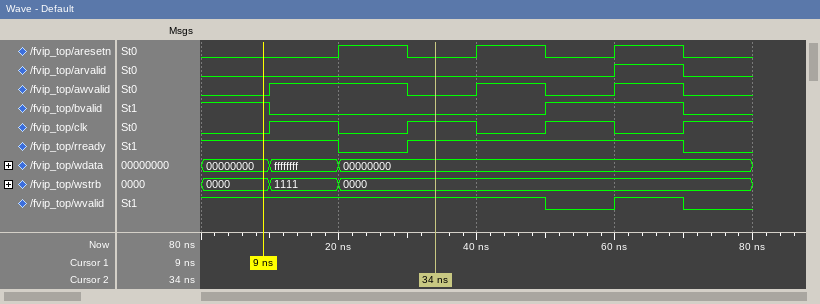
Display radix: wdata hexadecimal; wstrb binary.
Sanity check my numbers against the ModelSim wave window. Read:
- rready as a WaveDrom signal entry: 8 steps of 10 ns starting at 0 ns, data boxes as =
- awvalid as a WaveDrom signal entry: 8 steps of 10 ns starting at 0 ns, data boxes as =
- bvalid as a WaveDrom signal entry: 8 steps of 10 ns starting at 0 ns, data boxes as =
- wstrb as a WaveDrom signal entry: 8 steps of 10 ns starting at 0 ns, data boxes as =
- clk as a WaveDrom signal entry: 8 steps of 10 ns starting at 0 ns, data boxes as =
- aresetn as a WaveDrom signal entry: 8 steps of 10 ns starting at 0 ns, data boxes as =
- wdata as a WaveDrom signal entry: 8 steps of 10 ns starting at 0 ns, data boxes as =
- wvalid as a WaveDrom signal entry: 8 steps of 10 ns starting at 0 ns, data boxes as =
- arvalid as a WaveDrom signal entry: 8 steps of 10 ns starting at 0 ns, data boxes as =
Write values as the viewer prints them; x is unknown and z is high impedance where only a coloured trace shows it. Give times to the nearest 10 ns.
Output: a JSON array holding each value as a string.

["{name: 'rready', wave: '1.01...0'}", "{name: 'awvalid', wave: '01.01010'}", "{name: 'bvalid', wave: '10...1.0'}", "{name: 'wstrb', wave: '===.....', data: '0000 1111 0000'}", "{name: 'clk', wave: '01010101'}", "{name: 'aresetn', wave: '0.101010'}", "{name: 'wdata', wave: '===.....', data: '00000000 ffffffff 00000000'}", "{name: 'wvalid', wave: '1....010'}", "{name: 'arvalid', wave: '0.....10'}"]
